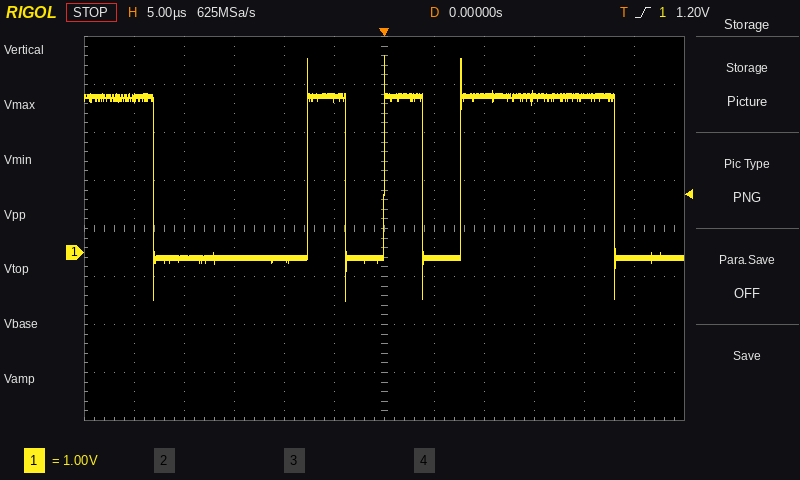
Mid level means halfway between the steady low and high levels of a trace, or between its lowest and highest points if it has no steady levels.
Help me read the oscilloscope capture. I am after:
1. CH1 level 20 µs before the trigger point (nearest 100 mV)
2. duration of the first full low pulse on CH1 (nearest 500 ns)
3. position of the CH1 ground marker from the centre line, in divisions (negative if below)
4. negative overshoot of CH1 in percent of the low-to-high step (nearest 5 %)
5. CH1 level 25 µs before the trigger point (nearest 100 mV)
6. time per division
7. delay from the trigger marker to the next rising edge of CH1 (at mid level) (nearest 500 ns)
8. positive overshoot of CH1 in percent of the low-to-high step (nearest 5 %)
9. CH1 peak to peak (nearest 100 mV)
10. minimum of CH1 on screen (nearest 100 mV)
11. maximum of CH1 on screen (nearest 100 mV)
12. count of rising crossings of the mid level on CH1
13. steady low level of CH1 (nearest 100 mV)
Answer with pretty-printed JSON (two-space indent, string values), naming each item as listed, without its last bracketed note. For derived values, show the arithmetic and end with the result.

{
  "CH1 level 20 µs before the trigger point": "-100 mV",
  "duration of the first full low pulse on CH1": "15.5 µs",
  "position of the CH1 ground marker from the centre line, in divisions": "-0.5 div",
  "negative overshoot of CH1 in percent of the low-to-high step": "25 %",
  "CH1 level 25 µs before the trigger point": "3.2 V",
  "time per division": "5 µs",
  "delay from the trigger marker to the next rising edge of CH1 (at mid level)": "7.5 µs",
  "positive overshoot of CH1 in percent of the low-to-high step": "25 %",
  "CH1 peak to peak": "4.1 V − (-1.0 V) = 5.1 V",
  "minimum of CH1 on screen": "-1.0 V",
  "maximum of CH1 on screen": "4.1 V",
  "count of rising crossings of the mid level on CH1": "3",
  "steady low level of CH1": "-100 mV"
}
